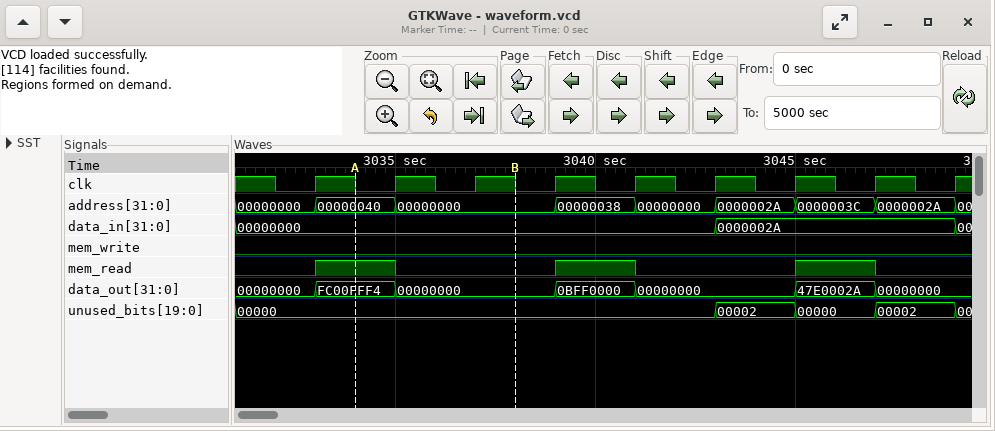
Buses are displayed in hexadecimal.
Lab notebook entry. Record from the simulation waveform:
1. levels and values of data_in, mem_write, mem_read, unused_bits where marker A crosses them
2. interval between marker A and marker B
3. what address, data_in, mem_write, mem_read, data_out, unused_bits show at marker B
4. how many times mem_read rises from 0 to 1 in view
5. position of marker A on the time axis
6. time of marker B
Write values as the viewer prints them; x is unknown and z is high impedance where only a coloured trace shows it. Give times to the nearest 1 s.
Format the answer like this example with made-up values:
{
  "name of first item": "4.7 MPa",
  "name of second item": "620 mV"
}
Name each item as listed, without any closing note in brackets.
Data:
{
  "levels and values of data_in, mem_write, mem_read, unused_bits where marker A crosses them": "data_in=00000000, mem_write=0, mem_read=1, unused_bits=00000",
  "interval between marker A and marker B": "4 s",
  "what address, data_in, mem_write, mem_read, data_out, unused_bits show at marker B": "address=00000000, data_in=00000000, mem_write=0, mem_read=0, data_out=00000000, unused_bits=00000",
  "how many times mem_read rises from 0 to 1 in view": "3",
  "position of marker A on the time axis": "3034 s",
  "time of marker B": "3038 s"
}
